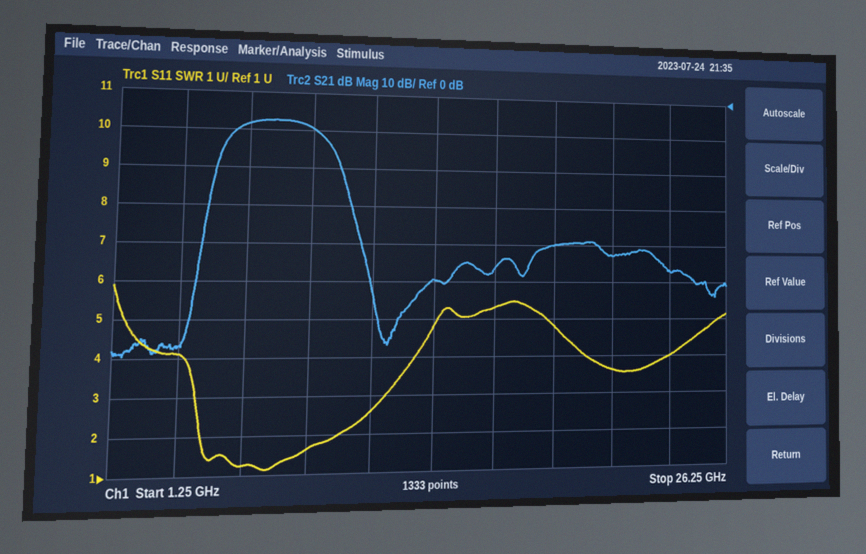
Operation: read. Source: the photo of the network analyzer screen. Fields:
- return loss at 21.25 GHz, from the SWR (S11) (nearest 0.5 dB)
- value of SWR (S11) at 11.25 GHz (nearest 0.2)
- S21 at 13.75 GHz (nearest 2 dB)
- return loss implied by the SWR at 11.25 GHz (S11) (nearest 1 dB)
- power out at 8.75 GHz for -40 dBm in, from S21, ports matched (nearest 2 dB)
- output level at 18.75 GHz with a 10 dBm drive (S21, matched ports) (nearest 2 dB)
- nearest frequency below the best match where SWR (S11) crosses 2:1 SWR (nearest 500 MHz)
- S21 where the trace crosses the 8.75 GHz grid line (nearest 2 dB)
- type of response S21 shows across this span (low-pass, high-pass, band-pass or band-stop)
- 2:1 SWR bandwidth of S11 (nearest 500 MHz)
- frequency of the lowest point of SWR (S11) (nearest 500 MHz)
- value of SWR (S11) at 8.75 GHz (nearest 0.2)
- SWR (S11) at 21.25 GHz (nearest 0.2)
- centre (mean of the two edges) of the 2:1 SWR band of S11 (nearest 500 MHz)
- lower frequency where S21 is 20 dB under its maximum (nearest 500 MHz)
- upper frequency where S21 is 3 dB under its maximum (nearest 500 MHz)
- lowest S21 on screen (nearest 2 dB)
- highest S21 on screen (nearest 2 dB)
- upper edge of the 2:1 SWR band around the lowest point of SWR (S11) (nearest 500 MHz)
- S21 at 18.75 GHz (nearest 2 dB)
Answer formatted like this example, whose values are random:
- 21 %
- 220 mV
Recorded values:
- 5.0 dB
- 2.6
- -50 dB
- 7 dB
- -50 dBm
- -30 dBm
- 4.5 GHz
- -10 dB
- band-pass
- 5.5 GHz
- 7.0 GHz
- 1.6
- 3.6
- 7.5 GHz
- 5.0 GHz
- 9.0 GHz
- -70 dB
- -8 dB
- 10.0 GHz
- -40 dB
